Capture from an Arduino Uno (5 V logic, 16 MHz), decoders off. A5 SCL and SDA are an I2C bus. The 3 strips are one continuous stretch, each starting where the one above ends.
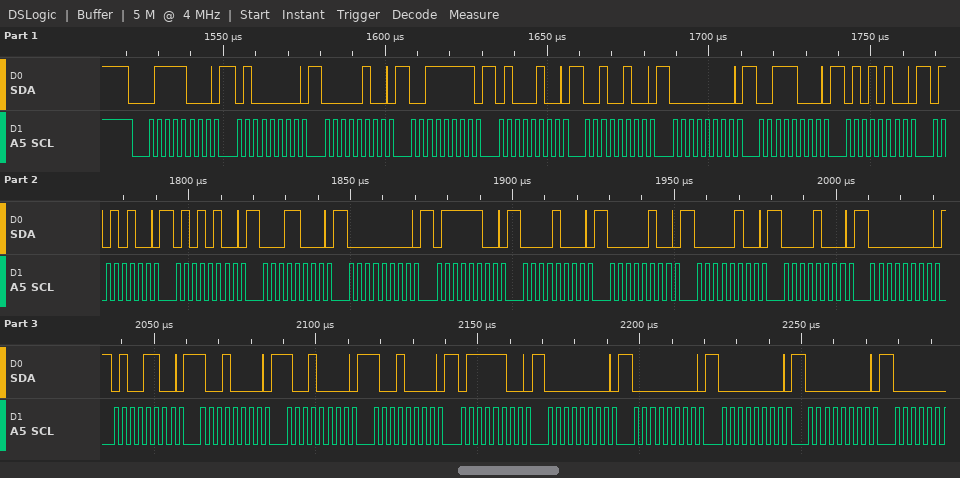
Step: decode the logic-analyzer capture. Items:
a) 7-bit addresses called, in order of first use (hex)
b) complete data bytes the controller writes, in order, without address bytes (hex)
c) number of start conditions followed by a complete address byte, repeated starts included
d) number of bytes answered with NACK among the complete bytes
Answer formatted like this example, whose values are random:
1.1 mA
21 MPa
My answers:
0x3C
40 04 3F 44 24 00 38 54 54 54 18 00 7C 08 04 04 08 00 4C 90 90 90 7C 00 00 00 00
1
0
